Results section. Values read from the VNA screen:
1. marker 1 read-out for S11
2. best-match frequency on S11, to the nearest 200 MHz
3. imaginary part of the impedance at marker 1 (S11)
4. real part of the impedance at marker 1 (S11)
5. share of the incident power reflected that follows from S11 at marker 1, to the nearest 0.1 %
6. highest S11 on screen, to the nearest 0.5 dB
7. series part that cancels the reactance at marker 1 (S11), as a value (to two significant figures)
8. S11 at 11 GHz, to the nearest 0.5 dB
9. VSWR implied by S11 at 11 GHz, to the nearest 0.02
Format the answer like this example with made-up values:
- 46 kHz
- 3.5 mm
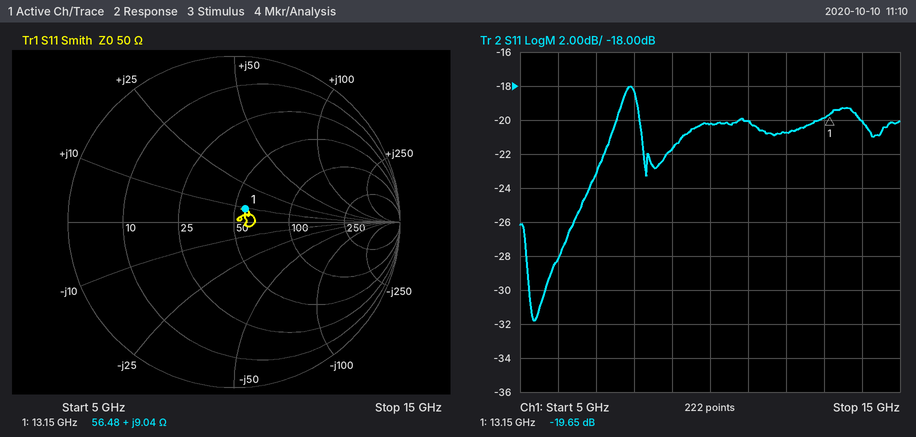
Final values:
- -19.65 dB
- 5.4 GHz
- +9.04 Ω
- 56.48 Ω
- 1.1 %
- -18.0 dB
- 1.3 pF
- -20.0 dB
- 1.22
